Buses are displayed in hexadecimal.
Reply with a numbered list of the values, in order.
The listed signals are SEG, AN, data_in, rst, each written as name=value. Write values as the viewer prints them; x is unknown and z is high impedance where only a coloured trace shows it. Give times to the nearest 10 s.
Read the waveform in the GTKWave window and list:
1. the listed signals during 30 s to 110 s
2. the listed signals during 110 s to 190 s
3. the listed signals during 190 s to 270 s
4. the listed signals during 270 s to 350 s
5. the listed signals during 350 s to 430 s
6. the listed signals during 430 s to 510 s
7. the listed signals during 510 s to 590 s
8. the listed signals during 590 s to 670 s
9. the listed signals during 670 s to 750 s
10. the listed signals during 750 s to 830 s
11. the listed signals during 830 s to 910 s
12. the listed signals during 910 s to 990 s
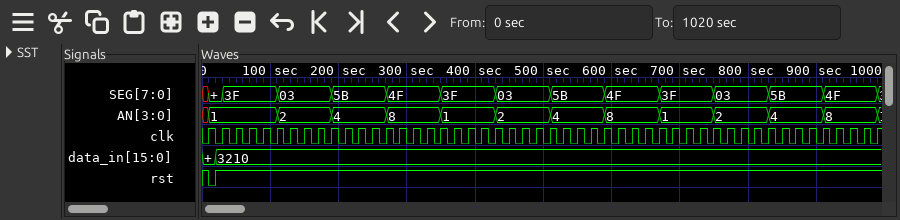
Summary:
1. SEG=3F, AN=1, data_in=3210, rst=1
2. SEG=03, AN=2, data_in=3210, rst=1
3. SEG=5B, AN=4, data_in=3210, rst=1
4. SEG=4F, AN=8, data_in=3210, rst=1
5. SEG=3F, AN=1, data_in=3210, rst=1
6. SEG=03, AN=2, data_in=3210, rst=1
7. SEG=5B, AN=4, data_in=3210, rst=1
8. SEG=4F, AN=8, data_in=3210, rst=1
9. SEG=3F, AN=1, data_in=3210, rst=1
10. SEG=03, AN=2, data_in=3210, rst=1
11. SEG=5B, AN=4, data_in=3210, rst=1
12. SEG=4F, AN=8, data_in=3210, rst=1
